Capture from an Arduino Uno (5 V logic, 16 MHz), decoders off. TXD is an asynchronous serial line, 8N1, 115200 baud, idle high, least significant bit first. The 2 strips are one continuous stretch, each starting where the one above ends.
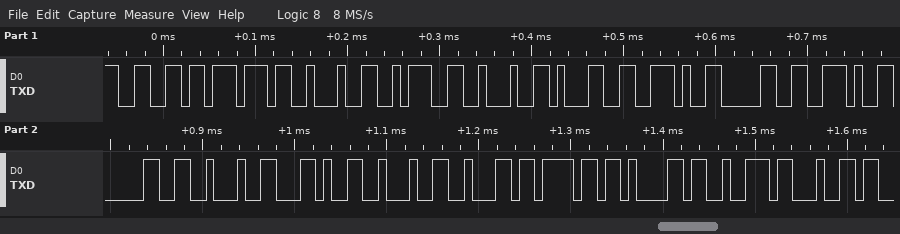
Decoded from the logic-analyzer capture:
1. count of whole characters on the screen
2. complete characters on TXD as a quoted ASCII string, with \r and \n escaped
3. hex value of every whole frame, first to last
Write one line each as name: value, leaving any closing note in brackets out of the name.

count of whole characters on the screen: 18
complete characters on TXD as a quoted ASCII string, with \r and \n escaped: "fw\":\"1.0.0\",\"board"
hex value of every whole frame, first to last: 66 77 22 3A 22 31 2E 30 2E 30 22 2C 22 62 6F 61 72 64
